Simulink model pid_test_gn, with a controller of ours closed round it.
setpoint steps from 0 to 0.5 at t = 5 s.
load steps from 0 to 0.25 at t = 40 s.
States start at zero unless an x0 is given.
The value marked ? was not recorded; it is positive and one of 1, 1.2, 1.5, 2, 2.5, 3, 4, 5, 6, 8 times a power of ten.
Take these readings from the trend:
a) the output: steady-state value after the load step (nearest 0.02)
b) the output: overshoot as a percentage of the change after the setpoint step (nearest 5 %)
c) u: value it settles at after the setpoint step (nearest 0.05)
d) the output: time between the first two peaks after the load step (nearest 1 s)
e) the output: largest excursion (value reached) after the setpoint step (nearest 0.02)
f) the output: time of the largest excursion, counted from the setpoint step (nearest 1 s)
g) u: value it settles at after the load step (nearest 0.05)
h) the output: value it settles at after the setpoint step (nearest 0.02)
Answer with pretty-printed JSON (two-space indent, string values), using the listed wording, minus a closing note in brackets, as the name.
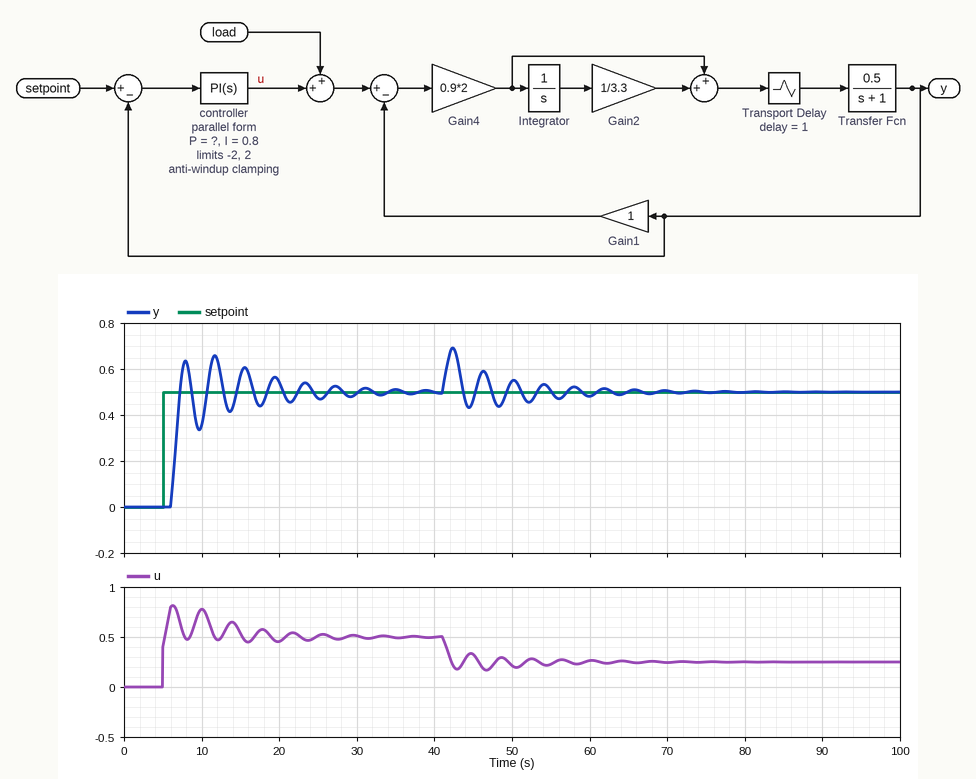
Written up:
{
  "the output: steady-state value after the load step": "0.50",
  "the output: overshoot as a percentage of the change after the setpoint step": "30 %",
  "u: value it settles at after the setpoint step": "0.50",
  "the output: time between the first two peaks after the load step": "4 s",
  "the output: largest excursion (value reached) after the setpoint step": "0.66",
  "the output: time of the largest excursion, counted from the setpoint step": "7 s",
  "u: value it settles at after the load step": "0.25",
  "the output: value it settles at after the setpoint step": "0.50"
}
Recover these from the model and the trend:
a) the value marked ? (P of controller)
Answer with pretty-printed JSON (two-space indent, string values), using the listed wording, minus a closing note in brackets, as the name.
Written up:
{
  "the value marked ?": "0.8"
}
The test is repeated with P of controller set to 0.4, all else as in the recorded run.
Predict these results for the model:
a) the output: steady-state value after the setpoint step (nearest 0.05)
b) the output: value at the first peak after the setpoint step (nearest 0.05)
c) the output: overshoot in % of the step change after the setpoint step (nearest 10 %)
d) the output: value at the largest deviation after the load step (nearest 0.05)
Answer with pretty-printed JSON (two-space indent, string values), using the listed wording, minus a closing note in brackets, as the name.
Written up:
{
  "the output: steady-state value after the setpoint step": "0.50",
  "the output: value at the first peak after the setpoint step": "0.60",
  "the output: overshoot in % of the step change after the setpoint step": "20 %",
  "the output: value at the largest deviation after the load step": "0.70"
}
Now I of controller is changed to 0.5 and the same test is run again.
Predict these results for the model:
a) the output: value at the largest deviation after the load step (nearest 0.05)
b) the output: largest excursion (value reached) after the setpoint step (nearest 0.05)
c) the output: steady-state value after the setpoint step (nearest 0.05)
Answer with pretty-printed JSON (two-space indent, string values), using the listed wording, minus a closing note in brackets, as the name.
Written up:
{
  "the output: value at the largest deviation after the load step": "0.70",
  "the output: largest excursion (value reached) after the setpoint step": "0.55",
  "the output: steady-state value after the setpoint step": "0.50"
}
